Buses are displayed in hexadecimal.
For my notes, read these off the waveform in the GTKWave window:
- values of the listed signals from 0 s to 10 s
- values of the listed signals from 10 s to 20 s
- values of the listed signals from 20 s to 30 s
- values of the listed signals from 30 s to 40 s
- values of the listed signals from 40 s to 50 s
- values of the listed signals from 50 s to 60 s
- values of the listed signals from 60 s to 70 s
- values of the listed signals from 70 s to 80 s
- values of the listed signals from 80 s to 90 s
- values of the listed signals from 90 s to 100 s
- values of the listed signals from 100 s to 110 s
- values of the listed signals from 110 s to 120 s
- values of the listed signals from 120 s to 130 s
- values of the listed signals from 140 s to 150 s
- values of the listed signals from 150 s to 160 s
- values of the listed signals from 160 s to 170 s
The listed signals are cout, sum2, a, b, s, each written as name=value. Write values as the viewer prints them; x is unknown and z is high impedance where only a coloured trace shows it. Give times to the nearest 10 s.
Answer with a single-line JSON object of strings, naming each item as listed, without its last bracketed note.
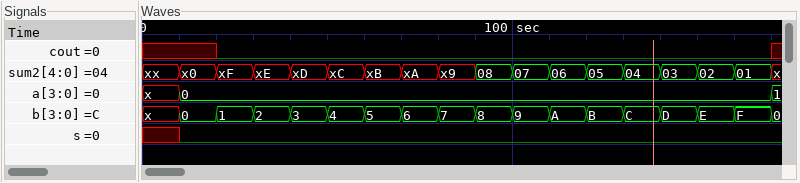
{"values of the listed signals from 0 s to 10 s": "cout=x, sum2=xx, a=x, b=x, s=x", "values of the listed signals from 10 s to 20 s": "cout=x, sum2=x0, a=0, b=0, s=0", "values of the listed signals from 20 s to 30 s": "cout=0, sum2=xF, a=0, b=1, s=0", "values of the listed signals from 30 s to 40 s": "cout=0, sum2=xE, a=0, b=2, s=0", "values of the listed signals from 40 s to 50 s": "cout=0, sum2=xD, a=0, b=3, s=0", "values of the listed signals from 50 s to 60 s": "cout=0, sum2=xC, a=0, b=4, s=0", "values of the listed signals from 60 s to 70 s": "cout=0, sum2=xB, a=0, b=5, s=0", "values of the listed signals from 70 s to 80 s": "cout=0, sum2=xA, a=0, b=6, s=0", "values of the listed signals from 80 s to 90 s": "cout=0, sum2=x9, a=0, b=7, s=0", "values of the listed signals from 90 s to 100 s": "cout=0, sum2=08, a=0, b=8, s=0", "values of the listed signals from 100 s to 110 s": "cout=0, sum2=07, a=0, b=9, s=0", "values of the listed signals from 110 s to 120 s": "cout=0, sum2=06, a=0, b=A, s=0", "values of the listed signals from 120 s to 130 s": "cout=0, sum2=05, a=0, b=B, s=0", "values of the listed signals from 140 s to 150 s": "cout=0, sum2=03, a=0, b=D, s=0", "values of the listed signals from 150 s to 160 s": "cout=0, sum2=02, a=0, b=E, s=0", "values of the listed signals from 160 s to 170 s": "cout=0, sum2=01, a=0, b=F, s=0"}
